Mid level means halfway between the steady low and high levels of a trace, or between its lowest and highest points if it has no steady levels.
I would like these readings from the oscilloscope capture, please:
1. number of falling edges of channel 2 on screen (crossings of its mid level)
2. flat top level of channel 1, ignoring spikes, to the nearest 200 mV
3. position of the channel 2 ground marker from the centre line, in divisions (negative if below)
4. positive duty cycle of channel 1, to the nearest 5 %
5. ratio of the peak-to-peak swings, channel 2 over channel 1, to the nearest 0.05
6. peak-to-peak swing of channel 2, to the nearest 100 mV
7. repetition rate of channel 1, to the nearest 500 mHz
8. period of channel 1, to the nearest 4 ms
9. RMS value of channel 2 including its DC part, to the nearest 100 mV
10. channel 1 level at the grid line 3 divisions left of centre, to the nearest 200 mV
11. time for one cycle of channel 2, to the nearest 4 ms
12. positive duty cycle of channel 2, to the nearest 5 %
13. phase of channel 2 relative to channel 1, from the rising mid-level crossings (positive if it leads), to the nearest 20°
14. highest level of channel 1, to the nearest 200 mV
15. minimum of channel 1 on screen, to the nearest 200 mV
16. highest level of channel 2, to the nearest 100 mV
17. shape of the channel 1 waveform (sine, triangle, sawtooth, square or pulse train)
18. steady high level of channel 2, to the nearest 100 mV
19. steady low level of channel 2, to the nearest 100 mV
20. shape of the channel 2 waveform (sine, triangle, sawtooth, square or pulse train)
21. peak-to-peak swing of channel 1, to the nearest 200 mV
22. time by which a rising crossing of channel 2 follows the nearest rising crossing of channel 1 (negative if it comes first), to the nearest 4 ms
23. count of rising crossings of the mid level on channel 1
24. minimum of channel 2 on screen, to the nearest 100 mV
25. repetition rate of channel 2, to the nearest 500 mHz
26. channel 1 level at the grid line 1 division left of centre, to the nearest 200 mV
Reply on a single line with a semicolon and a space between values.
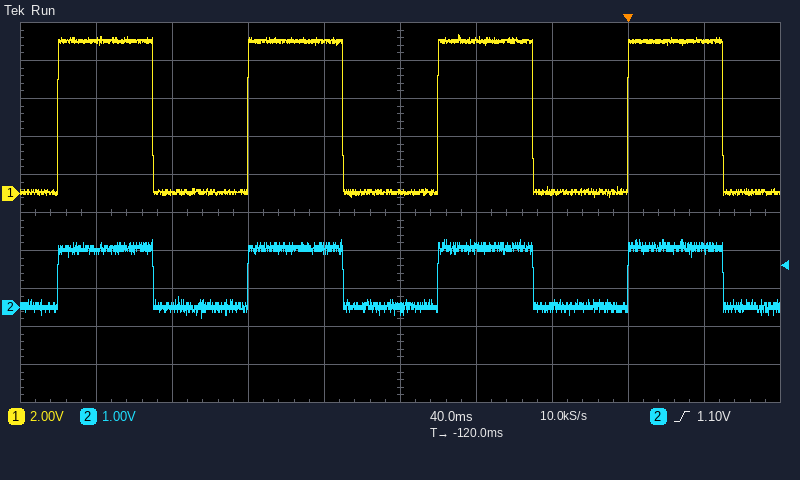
4; 8.0 V; -2.5 div; 50 %; 0.25; 2.1 V; 10.0 Hz; 100 ms; 1.1 V; 0.0 V; 100 ms; 50 %; 0°; 8.4 V; -200 mV; 1.8 V; square; 1.6 V; 0.0 V; square; 8.6 V; 0 ms; 4; -300 mV; 10.0 Hz; 8.0 V
